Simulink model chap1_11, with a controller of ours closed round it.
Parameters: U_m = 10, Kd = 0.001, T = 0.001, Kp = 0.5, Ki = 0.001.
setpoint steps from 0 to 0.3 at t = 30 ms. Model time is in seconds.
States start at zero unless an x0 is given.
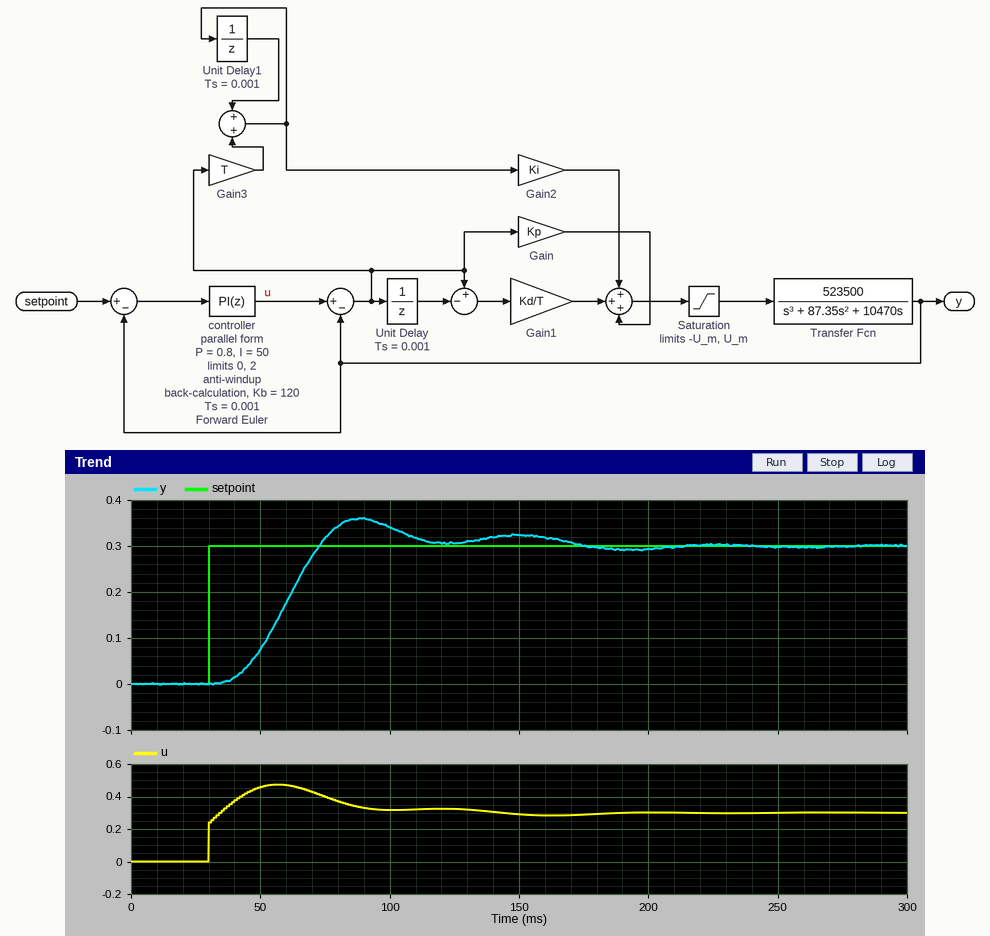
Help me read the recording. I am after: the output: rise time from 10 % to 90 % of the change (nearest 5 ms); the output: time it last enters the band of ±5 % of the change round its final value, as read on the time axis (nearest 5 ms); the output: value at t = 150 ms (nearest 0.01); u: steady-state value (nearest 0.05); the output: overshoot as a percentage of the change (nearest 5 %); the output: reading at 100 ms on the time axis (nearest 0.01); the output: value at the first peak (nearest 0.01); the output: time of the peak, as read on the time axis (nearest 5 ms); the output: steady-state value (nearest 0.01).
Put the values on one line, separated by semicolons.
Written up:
25 ms; 165 ms; 0.32; 0.30; 20 %; 0.34; 0.36; 90 ms; 0.30
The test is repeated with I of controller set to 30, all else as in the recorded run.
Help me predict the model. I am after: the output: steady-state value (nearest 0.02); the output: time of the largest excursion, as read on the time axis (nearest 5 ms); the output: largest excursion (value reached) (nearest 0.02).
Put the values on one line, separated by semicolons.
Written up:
0.30; 150 ms; 0.32
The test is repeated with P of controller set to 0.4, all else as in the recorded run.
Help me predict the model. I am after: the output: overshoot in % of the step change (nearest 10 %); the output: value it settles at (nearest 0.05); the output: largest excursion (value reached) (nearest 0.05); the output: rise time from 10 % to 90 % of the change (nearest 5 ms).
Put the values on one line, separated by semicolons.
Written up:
30 %; 0.30; 0.40; 30 ms
